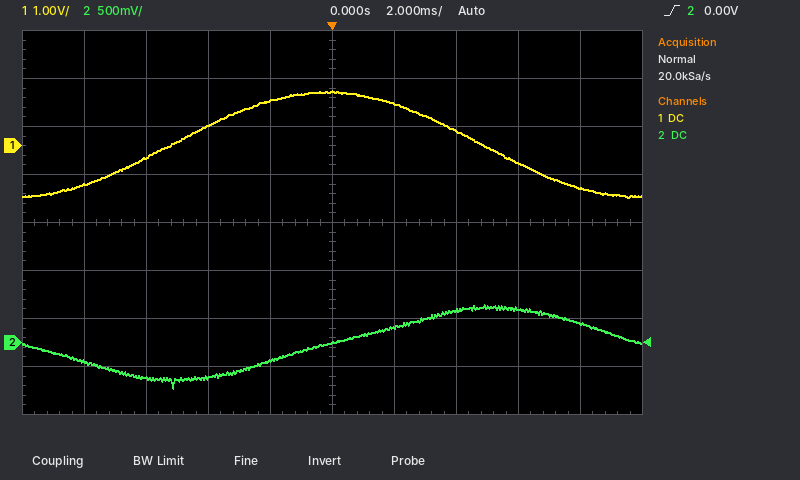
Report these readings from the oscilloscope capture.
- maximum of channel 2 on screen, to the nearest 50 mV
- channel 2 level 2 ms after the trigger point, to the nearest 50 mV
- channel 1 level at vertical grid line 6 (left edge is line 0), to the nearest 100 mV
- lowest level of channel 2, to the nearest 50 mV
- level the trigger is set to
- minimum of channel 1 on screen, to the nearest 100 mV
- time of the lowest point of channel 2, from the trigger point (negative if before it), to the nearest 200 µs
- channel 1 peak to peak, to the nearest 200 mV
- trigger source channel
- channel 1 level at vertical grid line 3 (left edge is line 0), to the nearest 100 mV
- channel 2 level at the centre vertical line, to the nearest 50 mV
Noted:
400 mV
150 mV
900 mV
-500 mV
0.00 V
-1.1 V
-5.2 ms
2.2 V
channel 2
400 mV
0 mV
